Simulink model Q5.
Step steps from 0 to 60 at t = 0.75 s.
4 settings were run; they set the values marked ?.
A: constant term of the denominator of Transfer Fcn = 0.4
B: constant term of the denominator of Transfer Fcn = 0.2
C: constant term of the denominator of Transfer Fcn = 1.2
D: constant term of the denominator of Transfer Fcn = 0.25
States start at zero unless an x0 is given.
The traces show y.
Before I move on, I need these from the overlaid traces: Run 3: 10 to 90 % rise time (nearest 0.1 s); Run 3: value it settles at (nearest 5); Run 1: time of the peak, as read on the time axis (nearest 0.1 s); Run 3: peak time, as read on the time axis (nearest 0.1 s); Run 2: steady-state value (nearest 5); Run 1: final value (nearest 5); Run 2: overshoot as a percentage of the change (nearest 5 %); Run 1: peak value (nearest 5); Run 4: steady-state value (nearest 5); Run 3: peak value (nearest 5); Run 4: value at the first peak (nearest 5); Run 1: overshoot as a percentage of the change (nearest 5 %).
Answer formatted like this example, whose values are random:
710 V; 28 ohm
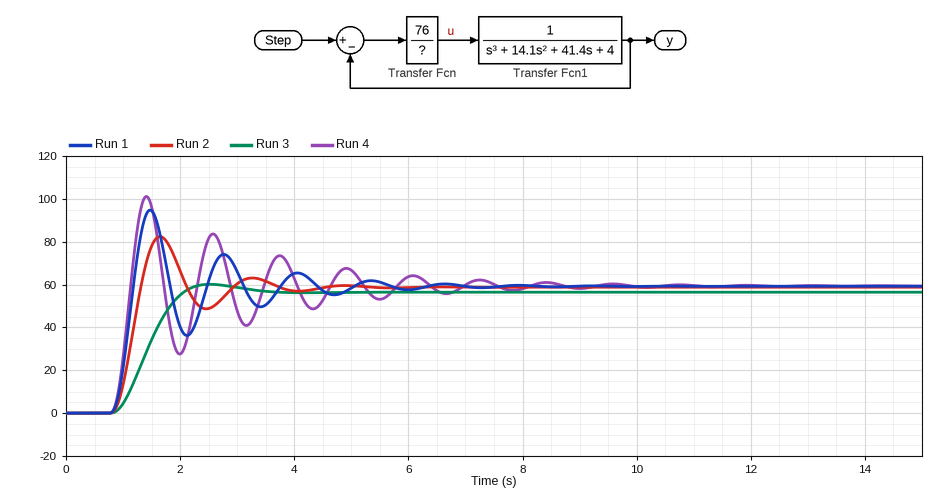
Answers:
0.8 s; 55; 1.5 s; 2.5 s; 60; 60; 40 %; 95; 60; 60; 100; 60 %
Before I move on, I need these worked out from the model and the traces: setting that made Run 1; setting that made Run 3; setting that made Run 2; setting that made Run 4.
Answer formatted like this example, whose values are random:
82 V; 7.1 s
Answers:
D; C; A; B
